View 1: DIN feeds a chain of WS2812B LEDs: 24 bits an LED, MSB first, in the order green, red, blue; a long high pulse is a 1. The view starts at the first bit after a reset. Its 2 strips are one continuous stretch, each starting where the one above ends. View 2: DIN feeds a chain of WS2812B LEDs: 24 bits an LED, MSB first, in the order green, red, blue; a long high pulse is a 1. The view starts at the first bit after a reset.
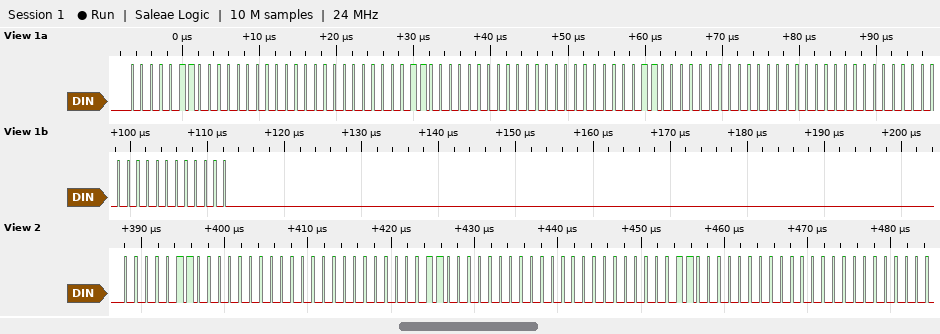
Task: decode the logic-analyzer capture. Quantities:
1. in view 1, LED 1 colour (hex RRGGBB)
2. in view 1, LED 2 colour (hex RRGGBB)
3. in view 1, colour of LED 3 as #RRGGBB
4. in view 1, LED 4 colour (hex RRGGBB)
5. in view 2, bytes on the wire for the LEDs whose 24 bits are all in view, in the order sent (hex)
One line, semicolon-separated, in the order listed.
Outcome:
#000600; #000600; #000600; #000000; 06 00 00 06 00 00 06 00 00
